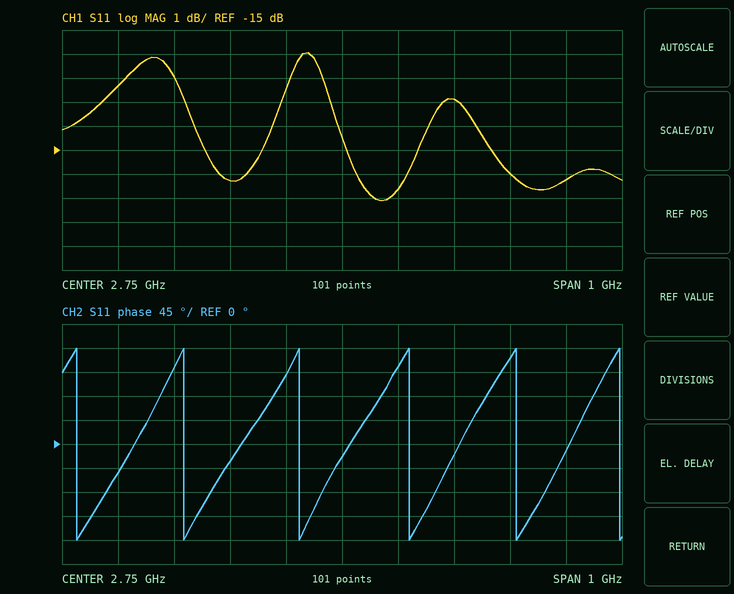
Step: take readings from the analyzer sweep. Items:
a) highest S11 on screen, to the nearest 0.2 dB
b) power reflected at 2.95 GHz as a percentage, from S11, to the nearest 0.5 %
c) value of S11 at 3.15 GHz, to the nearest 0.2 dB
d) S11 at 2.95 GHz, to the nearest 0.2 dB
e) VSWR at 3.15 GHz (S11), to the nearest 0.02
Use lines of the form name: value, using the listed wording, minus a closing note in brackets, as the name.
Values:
highest S11 on screen, to the nearest 0.2 dB: -11.0 dB
power reflected at 2.95 GHz as a percentage, from S11, to the nearest 0.5 %: 5.0 %
value of S11 at 3.15 GHz, to the nearest 0.2 dB: -16.2 dB
S11 at 2.95 GHz, to the nearest 0.2 dB: -12.8 dB
VSWR at 3.15 GHz (S11), to the nearest 0.02: 1.36
